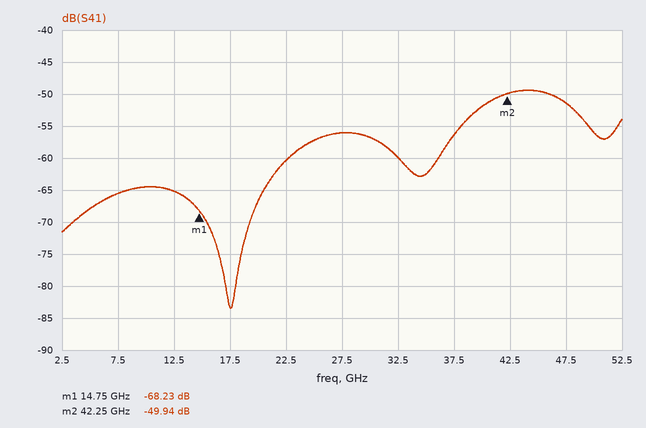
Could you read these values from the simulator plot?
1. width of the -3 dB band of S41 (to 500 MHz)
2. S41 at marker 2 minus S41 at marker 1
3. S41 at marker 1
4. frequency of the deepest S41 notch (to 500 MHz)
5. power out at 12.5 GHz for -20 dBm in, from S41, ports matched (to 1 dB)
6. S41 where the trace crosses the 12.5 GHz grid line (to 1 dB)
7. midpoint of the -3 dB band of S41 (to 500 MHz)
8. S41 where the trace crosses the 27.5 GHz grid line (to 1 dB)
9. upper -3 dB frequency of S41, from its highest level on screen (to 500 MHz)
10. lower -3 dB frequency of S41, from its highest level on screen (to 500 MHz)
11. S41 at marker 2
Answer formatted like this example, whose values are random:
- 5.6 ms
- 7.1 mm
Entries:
- 8.5 GHz
- 18.29 dB
- -68.23 dB
- 17.5 GHz
- -85 dBm
- -65 dB
- 44.0 GHz
- -56 dB
- 48.0 GHz
- 39.5 GHz
- -49.94 dB
